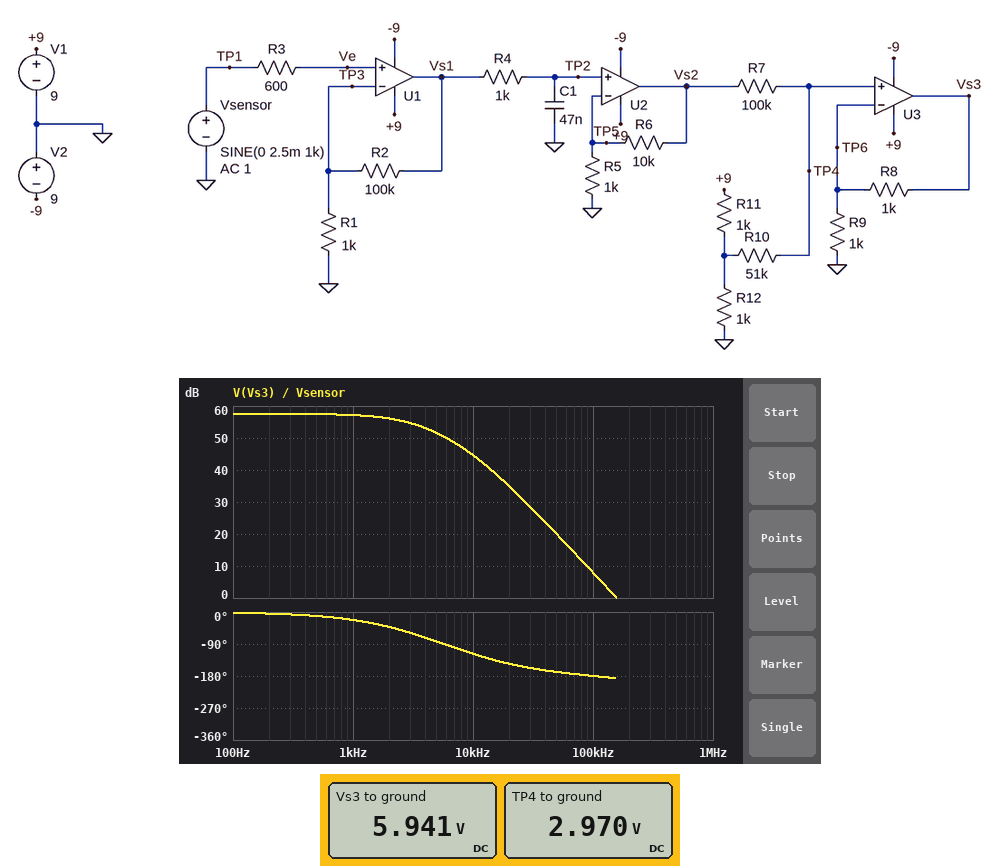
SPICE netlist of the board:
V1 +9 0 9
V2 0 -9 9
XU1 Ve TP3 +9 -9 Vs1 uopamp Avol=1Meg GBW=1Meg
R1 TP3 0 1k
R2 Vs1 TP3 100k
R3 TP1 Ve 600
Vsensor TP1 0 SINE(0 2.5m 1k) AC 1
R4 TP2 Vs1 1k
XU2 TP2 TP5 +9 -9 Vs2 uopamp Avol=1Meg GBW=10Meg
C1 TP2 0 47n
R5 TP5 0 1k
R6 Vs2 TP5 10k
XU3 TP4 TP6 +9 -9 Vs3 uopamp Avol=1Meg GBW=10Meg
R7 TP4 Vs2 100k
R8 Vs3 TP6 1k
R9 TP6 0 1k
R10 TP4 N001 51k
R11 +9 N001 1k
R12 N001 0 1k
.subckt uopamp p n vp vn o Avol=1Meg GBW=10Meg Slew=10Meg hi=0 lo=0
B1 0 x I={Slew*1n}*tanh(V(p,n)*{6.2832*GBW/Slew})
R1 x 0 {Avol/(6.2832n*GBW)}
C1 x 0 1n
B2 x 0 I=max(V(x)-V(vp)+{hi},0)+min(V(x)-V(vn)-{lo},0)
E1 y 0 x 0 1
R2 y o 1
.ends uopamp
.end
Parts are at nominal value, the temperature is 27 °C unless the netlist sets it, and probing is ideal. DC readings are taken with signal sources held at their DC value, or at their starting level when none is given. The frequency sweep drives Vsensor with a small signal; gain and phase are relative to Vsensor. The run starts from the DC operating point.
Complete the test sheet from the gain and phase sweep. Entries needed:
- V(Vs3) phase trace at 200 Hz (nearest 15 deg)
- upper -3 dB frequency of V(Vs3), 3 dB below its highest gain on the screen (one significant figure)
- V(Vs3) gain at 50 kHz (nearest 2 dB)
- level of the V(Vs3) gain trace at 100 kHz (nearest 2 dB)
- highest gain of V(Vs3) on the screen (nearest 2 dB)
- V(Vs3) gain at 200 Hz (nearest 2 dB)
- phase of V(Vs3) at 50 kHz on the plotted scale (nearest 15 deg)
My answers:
0 deg
3 kHz
20 dB
8 dB
58 dB
58 dB
-165 deg
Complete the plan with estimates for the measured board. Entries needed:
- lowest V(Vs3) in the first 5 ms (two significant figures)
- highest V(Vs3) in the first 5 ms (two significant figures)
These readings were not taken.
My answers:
4.1 V
7.7 V
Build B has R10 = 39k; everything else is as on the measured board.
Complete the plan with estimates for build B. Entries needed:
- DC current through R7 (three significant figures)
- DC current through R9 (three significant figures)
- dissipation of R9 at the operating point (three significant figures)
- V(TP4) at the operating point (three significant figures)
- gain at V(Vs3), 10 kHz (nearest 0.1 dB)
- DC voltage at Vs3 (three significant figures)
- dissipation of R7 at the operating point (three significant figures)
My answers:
32.3 µA
3.23 mA
10.4 mW
3.23 V
43.0 dB
6.45 V
104 µW
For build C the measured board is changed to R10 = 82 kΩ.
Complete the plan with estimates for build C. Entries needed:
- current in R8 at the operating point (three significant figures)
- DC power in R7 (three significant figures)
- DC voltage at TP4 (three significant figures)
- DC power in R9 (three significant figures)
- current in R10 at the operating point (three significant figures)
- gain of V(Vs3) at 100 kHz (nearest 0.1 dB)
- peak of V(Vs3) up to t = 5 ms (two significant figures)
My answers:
2.47 mA
60.8 µW
2.47 V
6.08 mW
24.7 µA
10.4 dB
7.3 V
